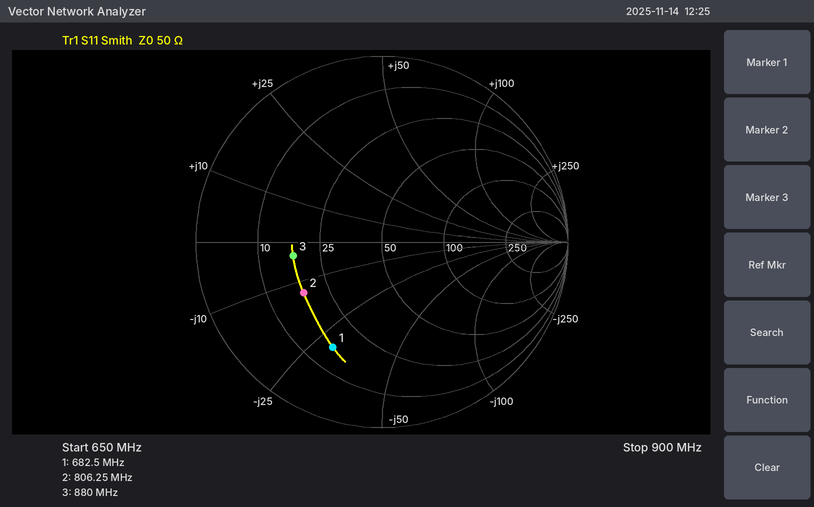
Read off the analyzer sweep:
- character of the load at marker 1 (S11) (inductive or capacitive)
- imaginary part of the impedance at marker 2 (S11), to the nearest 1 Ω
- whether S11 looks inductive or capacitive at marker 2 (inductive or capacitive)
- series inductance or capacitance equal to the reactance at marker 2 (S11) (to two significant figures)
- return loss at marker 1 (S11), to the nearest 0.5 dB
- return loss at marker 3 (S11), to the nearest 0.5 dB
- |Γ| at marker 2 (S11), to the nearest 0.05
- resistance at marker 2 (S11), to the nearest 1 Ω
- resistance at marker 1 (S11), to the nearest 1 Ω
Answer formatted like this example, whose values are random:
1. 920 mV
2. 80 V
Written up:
1. capacitive
2. -13 Ω
3. capacitive
4. 15 pF
5. 4.0 dB
6. 6.5 dB
7. 0.50
8. 18 Ω
9. 16 Ω
